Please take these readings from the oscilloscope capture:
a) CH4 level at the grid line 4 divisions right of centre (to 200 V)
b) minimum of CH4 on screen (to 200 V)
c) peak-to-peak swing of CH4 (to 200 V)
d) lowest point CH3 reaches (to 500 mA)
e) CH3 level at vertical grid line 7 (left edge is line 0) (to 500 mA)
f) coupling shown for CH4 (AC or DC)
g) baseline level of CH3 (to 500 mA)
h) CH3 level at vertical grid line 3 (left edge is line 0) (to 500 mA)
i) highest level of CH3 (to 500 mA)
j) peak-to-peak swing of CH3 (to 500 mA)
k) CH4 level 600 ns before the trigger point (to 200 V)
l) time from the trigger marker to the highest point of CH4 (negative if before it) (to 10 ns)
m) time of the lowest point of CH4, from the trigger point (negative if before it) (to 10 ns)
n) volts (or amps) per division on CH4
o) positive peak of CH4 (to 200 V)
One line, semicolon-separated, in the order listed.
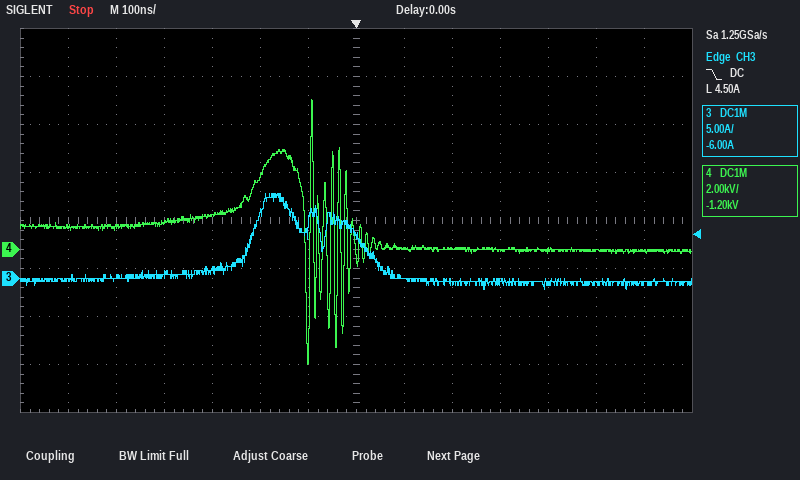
0.0 kV; -4.8 kV; 11.0 kV; -1.0 A; 4.5 A; DC; -500 mA; 500 mA; 9.0 A; 10.0 A; 1.0 kV; -90 ns; -100 ns; 2 kV; 6.2 kV
